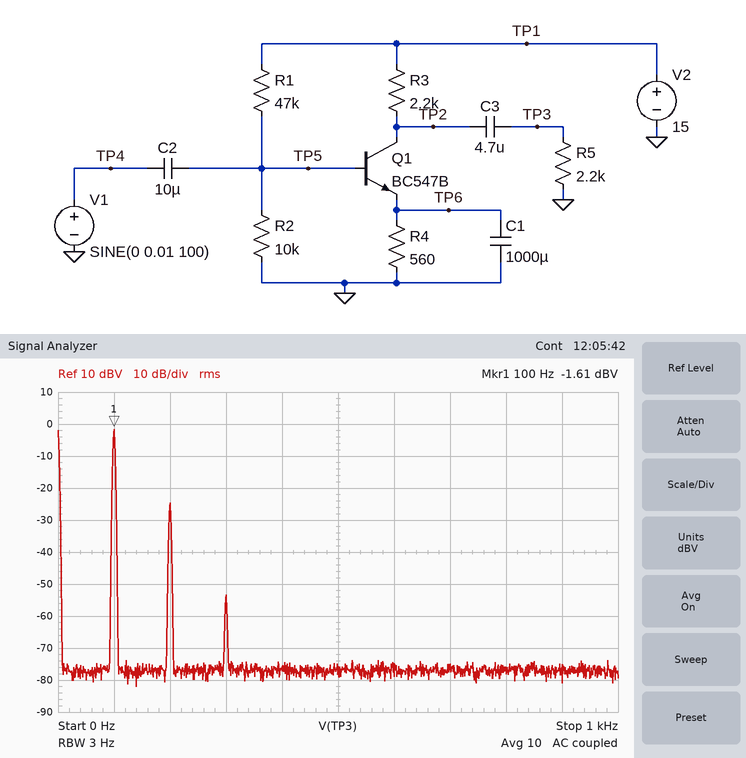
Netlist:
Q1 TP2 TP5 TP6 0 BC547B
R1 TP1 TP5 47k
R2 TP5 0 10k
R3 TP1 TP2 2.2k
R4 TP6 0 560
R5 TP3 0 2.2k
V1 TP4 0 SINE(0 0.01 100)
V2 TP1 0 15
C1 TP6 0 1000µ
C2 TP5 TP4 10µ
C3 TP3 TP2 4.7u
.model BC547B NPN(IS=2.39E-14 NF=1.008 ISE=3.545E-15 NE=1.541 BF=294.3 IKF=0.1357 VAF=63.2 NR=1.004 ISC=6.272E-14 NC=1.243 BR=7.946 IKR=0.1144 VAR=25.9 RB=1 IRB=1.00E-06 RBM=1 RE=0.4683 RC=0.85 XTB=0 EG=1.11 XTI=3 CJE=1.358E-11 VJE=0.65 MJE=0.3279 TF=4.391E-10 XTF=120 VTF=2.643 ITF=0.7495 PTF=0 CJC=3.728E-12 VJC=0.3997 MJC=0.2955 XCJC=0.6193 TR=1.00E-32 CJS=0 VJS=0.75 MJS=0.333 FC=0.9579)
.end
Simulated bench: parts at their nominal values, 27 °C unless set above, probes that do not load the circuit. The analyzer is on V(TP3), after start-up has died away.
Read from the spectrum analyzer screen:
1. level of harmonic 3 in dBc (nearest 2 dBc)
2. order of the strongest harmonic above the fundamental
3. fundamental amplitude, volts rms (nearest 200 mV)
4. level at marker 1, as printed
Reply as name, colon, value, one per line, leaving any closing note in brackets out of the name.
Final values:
level of harmonic 3 in dBc: -52 dBc
order of the strongest harmonic above the fundamental: 2
fundamental amplitude, volts rms: 800 mV
level at marker 1, as printed: -1.61 dBV
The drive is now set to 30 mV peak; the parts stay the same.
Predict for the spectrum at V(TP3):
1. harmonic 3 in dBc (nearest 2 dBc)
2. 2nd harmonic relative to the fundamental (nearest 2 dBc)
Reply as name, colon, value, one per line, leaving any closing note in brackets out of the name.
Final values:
harmonic 3 in dBc: -32 dBc
2nd harmonic relative to the fundamental: -14 dBc
